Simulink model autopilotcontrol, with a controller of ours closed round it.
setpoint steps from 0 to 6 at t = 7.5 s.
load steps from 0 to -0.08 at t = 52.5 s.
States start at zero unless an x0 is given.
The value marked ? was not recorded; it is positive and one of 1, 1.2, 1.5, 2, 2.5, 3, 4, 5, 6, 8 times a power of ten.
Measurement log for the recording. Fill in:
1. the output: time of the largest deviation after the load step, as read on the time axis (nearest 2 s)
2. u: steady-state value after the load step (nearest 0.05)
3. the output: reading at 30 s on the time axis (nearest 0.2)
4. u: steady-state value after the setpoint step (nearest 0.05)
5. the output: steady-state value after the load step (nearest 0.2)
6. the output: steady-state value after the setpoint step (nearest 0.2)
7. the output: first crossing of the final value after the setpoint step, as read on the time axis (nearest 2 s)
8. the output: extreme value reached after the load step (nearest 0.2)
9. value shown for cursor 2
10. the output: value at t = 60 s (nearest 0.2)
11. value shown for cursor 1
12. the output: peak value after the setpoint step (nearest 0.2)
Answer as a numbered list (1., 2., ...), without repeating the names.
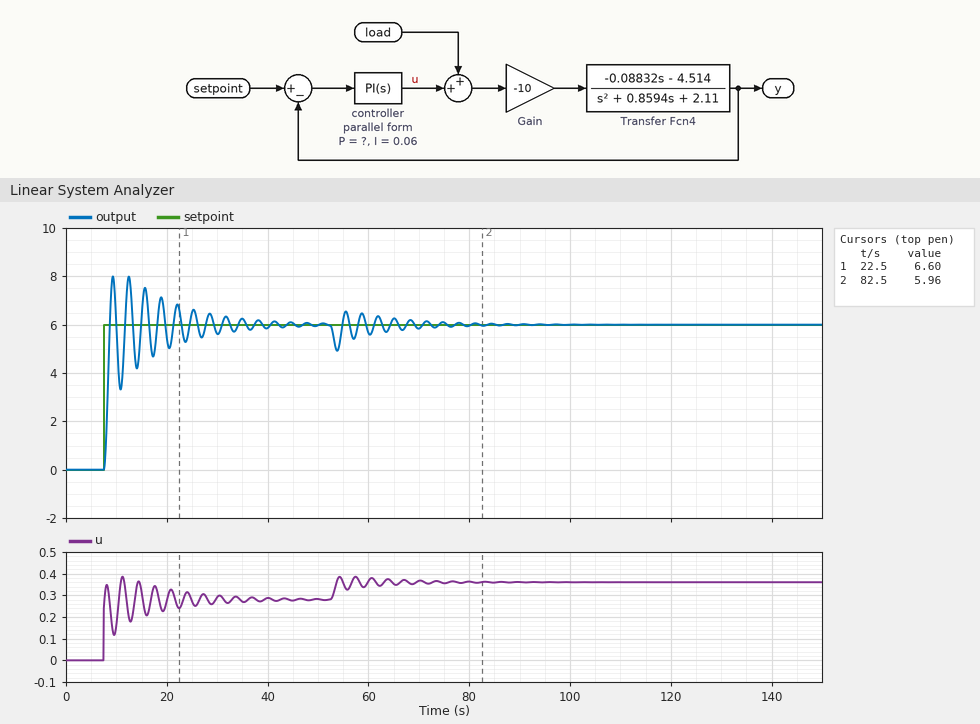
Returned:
1. 54 s
2. 0.35
3. 5.6
4. 0.30
5. 6.0
6. 6.0
7. 8 s
8. 5.0
9. 5.96
10. 5.6
11. 6.60
12. 8.0
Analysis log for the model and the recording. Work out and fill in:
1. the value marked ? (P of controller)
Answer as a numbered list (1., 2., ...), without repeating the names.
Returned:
1. 0.04
